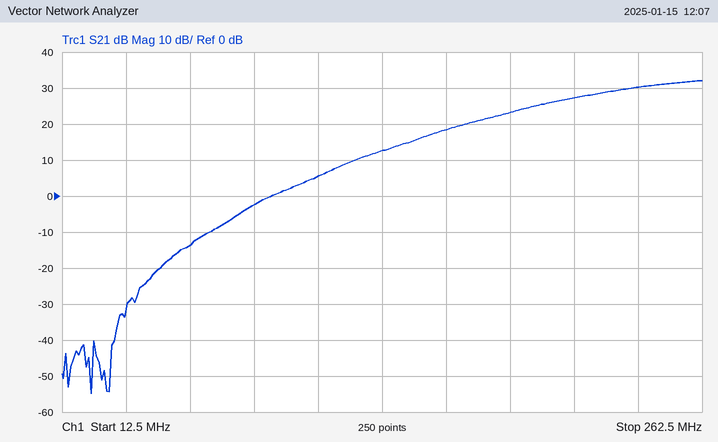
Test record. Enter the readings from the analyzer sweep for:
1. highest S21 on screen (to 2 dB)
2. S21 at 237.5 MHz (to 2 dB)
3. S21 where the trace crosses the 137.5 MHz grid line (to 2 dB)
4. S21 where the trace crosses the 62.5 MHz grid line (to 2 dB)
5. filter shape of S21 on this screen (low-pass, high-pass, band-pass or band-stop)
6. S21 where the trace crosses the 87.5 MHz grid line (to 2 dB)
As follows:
32 dB
30 dB
12 dB
-14 dB
high-pass
-2 dB
